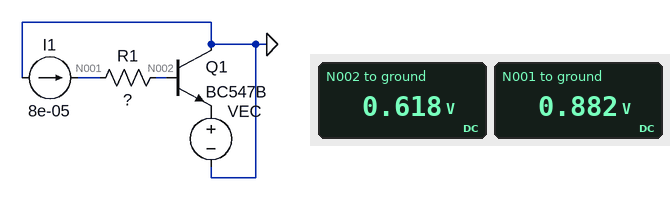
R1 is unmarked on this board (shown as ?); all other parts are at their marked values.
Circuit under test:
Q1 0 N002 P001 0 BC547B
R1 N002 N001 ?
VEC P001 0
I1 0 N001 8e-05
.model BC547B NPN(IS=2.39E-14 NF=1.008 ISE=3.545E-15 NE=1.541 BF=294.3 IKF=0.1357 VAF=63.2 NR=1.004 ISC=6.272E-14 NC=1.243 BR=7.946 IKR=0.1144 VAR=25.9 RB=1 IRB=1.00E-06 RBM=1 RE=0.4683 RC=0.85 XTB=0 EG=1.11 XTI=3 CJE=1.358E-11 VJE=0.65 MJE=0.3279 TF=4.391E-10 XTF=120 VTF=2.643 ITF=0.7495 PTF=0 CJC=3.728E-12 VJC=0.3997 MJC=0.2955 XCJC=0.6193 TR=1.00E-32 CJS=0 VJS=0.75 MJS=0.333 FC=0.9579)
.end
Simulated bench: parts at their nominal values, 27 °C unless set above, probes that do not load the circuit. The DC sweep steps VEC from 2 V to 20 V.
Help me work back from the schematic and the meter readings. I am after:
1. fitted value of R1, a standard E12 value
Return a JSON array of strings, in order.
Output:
["3.3 kΩ"]
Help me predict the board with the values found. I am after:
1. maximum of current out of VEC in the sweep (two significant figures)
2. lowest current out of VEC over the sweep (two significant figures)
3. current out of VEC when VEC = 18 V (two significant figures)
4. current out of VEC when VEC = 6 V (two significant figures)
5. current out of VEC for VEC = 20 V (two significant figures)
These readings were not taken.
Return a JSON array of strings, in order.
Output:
["910 µA", "540 µA", "870 µA", "620 µA", "910 µA"]
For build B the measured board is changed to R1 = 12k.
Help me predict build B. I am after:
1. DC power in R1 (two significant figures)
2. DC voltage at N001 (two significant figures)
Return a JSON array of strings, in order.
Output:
["77 µW", "1.6 V"]
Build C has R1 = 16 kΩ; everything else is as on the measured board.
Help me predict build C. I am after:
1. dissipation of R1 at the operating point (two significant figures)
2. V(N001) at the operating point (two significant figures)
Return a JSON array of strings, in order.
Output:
["100 µW", "1.9 V"]
